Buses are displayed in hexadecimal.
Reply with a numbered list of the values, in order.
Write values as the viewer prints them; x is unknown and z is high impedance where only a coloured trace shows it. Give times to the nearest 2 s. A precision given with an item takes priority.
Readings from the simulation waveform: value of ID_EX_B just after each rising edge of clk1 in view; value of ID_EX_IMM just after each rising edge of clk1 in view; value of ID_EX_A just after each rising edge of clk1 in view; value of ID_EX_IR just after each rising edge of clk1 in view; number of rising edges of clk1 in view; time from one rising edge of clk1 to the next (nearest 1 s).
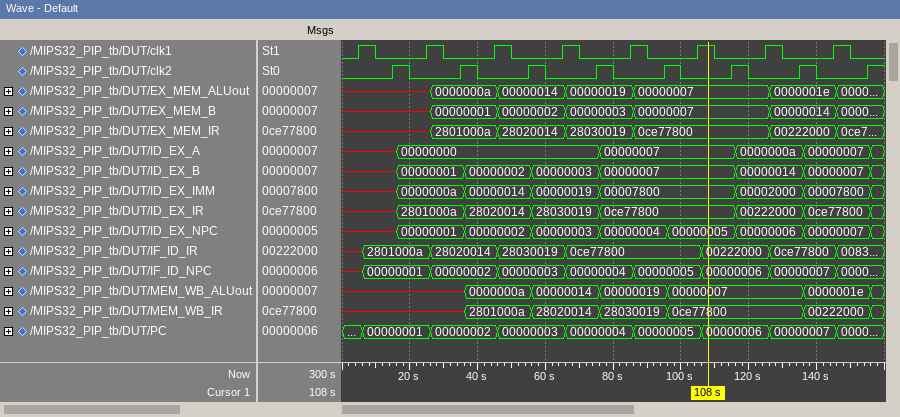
1. x, 00000001, 00000002, 00000003, 00000007, 00000007, 00000014, 00000007
2. x, 0000000a, 00000014, 00000019, 00007800, 00007800, 00002000, 00007800
3. x, 00000000, 00000000, 00000000, 00000007, 00000007, 0000000a, 00000007
4. x, 2801000a, 28020014, 28030019, 0ce77800, 0ce77800, 00222000, 0ce77800
5. 8
6. 20 s
